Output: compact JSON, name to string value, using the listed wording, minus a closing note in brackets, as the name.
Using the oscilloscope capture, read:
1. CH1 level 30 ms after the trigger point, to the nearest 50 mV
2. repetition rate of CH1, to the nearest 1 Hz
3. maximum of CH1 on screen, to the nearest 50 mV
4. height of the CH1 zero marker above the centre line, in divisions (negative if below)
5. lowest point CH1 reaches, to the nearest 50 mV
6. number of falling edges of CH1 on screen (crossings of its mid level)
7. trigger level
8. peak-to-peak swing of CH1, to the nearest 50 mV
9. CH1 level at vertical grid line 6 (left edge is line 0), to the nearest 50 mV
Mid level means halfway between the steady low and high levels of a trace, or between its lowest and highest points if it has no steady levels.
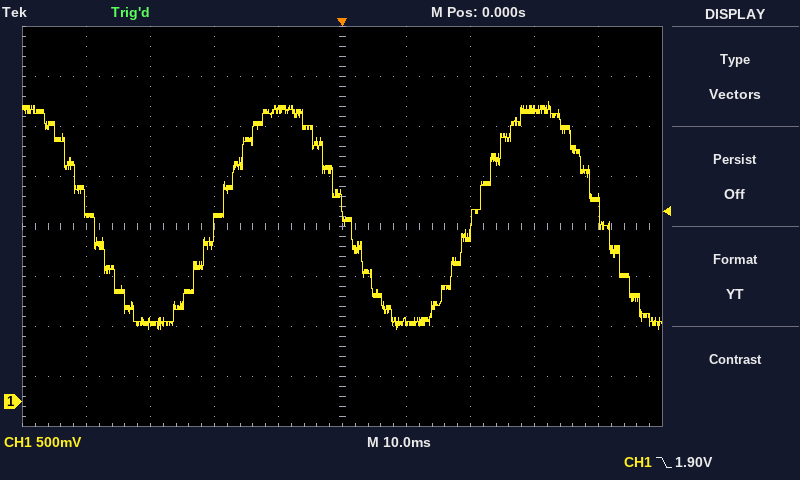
{"CH1 level 30 ms after the trigger point, to the nearest 50 mV": "2.90 V", "repetition rate of CH1, to the nearest 1 Hz": "25 Hz", "maximum of CH1 on screen, to the nearest 50 mV": "3.00 V", "height of the CH1 zero marker above the centre line, in divisions": "-3.5 div", "lowest point CH1 reaches, to the nearest 50 mV": "700 mV", "number of falling edges of CH1 on screen": "3", "trigger level": "1.90 V", "peak-to-peak swing of CH1, to the nearest 50 mV": "2.30 V", "CH1 level at vertical grid line 6 (left edge is line 0), to the nearest 50 mV": "800 mV"}
